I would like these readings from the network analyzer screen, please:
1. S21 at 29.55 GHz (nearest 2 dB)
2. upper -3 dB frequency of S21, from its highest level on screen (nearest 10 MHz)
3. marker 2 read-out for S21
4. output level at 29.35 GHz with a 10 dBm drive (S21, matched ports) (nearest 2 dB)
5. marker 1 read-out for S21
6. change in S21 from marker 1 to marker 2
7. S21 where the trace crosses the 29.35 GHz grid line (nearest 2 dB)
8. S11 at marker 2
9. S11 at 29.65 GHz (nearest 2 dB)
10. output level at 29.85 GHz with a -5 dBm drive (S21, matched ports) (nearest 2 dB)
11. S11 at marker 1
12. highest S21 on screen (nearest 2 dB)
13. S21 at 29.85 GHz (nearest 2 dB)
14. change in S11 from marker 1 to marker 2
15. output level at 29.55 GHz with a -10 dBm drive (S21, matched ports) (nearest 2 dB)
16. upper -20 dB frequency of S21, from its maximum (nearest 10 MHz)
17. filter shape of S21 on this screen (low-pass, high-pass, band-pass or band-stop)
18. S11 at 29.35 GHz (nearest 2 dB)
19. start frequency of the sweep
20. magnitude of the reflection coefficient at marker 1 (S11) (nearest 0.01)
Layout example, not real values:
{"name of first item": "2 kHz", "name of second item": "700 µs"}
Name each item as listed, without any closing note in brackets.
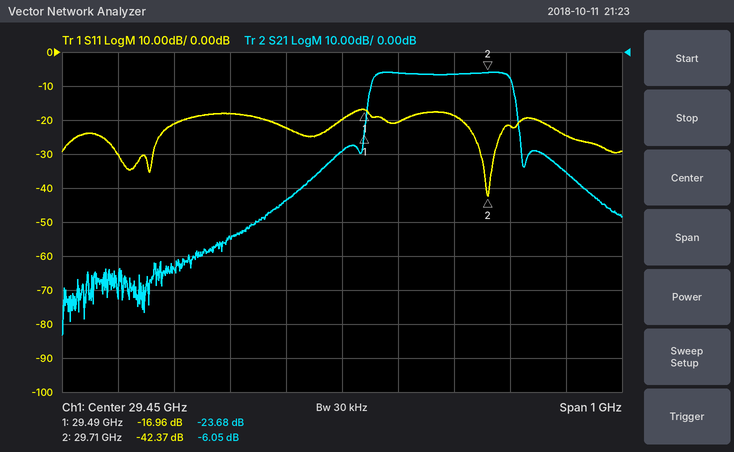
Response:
{"S21 at 29.55 GHz": "-6 dB", "upper -3 dB frequency of S21, from its highest level on screen": "29.75 GHz", "marker 2 read-out for S21": "-6.05 dB", "output level at 29.35 GHz with a 10 dBm drive (S21, matched ports)": "-34 dBm", "marker 1 read-out for S21": "-23.68 dB", "change in S21 from marker 1 to marker 2": "17.63 dB", "S21 where the trace crosses the 29.35 GHz grid line": "-44 dB", "S11 at marker 2": "-42.37 dB", "S11 at 29.65 GHz": "-18 dB", "output level at 29.85 GHz with a -5 dBm drive (S21, matched ports)": "-40 dBm", "S11 at marker 1": "-16.96 dB", "highest S21 on screen": "-6 dB", "S21 at 29.85 GHz": "-36 dB", "change in S11 from marker 1 to marker 2": "-25.41 dB", "output level at 29.55 GHz with a -10 dBm drive (S21, matched ports)": "-16 dBm", "upper -20 dB frequency of S21, from its maximum": "29.77 GHz", "filter shape of S21 on this screen": "band-pass", "S11 at 29.35 GHz": "-22 dB", "start frequency of the sweep": "28.95 GHz", "magnitude of the reflection coefficient at marker 1 (S11)": "0.14"}
